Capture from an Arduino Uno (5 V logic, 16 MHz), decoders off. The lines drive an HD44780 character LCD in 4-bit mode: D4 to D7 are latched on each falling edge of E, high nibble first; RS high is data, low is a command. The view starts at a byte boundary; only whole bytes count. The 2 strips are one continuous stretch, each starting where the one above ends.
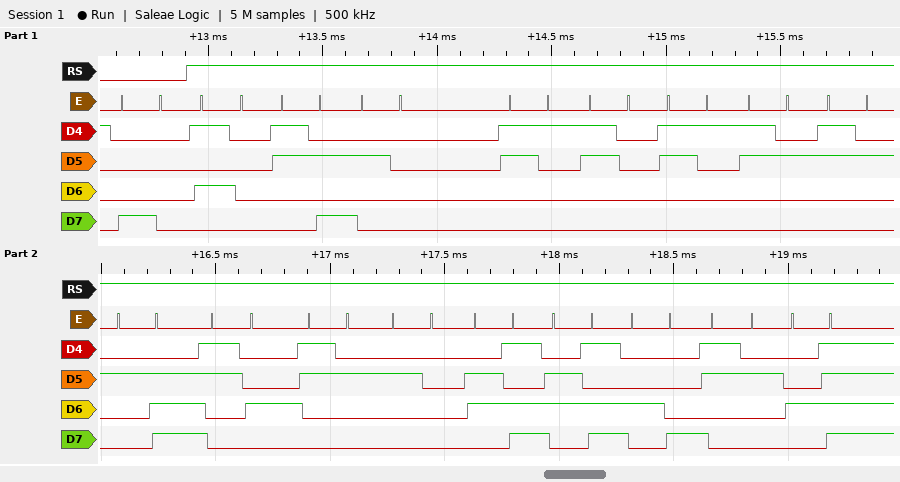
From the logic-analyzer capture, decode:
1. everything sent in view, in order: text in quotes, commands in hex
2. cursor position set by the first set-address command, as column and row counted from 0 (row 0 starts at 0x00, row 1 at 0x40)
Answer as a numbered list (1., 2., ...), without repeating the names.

1. 0x80 "P: 10122.42 mmH2O"
2. column 0, row 0
